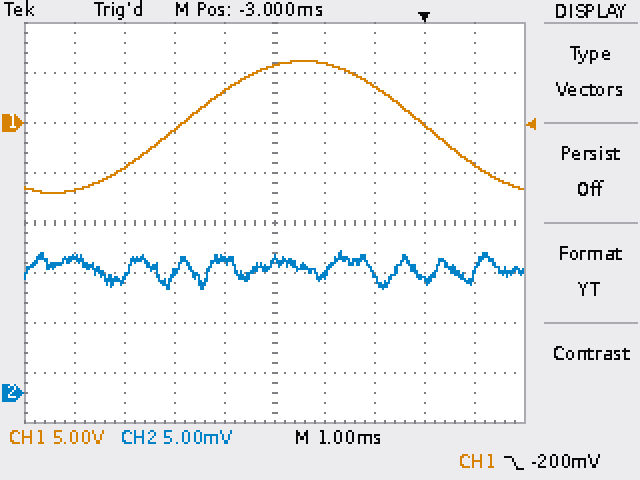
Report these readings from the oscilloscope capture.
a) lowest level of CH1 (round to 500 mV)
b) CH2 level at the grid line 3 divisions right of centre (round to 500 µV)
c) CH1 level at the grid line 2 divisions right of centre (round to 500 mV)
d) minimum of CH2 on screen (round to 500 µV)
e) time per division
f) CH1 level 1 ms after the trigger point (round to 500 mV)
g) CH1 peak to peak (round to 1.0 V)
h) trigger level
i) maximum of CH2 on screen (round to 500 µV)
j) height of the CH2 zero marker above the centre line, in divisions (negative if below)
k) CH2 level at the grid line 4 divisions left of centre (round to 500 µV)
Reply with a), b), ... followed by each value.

a) -7.0 V
b) 11.5 mV
c) 3.5 V
d) 10.5 mV
e) 1 ms
f) -4.0 V
g) 13.0 V
h) -200 mV
i) 14.0 mV
j) -3.4 div
k) 13.5 mV
